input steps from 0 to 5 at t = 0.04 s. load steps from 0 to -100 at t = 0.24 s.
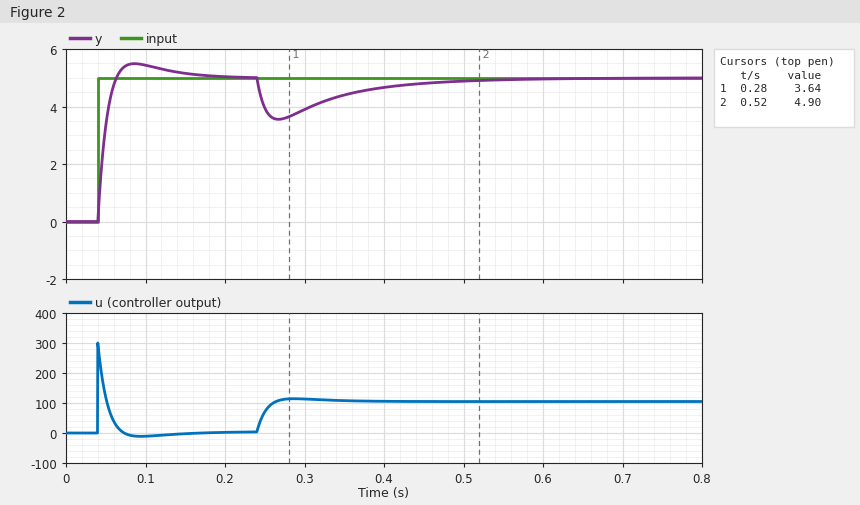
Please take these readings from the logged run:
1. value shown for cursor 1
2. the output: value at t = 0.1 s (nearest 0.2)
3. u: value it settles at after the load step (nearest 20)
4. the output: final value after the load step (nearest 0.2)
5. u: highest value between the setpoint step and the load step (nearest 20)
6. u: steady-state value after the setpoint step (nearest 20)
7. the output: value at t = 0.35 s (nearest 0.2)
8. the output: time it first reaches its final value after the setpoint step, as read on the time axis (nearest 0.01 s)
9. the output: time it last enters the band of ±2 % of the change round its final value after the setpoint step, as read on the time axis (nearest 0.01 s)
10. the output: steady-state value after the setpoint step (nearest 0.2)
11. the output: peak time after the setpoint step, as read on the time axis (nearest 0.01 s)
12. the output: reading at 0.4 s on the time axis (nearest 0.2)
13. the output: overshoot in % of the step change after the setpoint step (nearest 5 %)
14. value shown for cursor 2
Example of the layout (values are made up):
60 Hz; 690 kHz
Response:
3.64; 5.4; 100; 5.0; 300; 0; 4.4; 0.06 s; 0.17 s; 5.0; 0.09 s; 4.6; 10 %; 4.90
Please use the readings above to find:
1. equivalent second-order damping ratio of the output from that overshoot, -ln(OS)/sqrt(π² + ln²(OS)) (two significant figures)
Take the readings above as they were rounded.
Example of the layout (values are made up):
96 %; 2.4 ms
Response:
0.59
